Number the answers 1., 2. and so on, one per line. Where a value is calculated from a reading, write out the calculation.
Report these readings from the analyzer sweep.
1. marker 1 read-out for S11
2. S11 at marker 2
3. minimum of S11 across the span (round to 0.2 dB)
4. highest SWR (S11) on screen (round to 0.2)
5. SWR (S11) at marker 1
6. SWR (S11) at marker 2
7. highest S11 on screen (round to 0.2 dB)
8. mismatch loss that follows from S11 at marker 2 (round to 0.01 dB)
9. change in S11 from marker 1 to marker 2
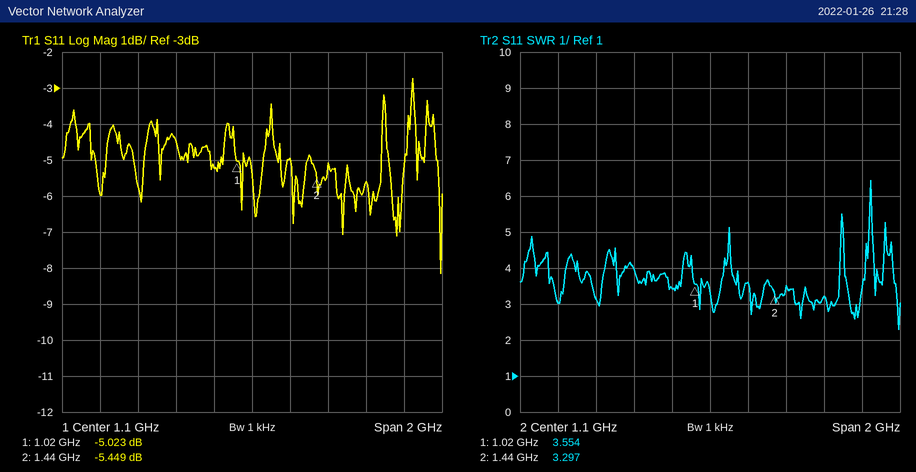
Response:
1. -5.023 dB
2. -5.449 dB
3. -8.2 dB
4. 6.4
5. 3.554
6. 3.297
7. -2.8 dB
8. −10 log10(1 − 10^(-5.449/10)) ≈ 1.46 dB
9. -5.449 − (-5.023) = -0.426 dB
